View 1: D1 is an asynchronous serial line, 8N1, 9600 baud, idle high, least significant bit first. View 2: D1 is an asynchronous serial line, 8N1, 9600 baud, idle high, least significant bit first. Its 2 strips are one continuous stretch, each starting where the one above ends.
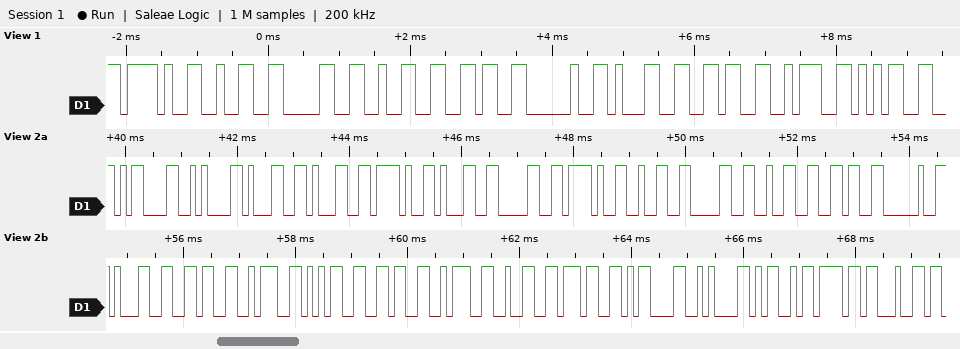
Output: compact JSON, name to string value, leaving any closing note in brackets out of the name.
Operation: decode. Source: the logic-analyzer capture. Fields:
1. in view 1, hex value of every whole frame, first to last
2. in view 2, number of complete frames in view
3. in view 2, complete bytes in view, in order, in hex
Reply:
{"in view 1, hex value of every whole frame, first to last": "2F 32 30 32 36 20 31 36 3A 35", "in view 2, number of complete frames in view": "26", "in view 2, complete bytes in view, in order, in hex": "0D 0A 31 31 2F 31 30 2F 32 30 32 36 20 31 36 3A 35 36 3A 32 37 0D 0A 4D 6F 64"}
